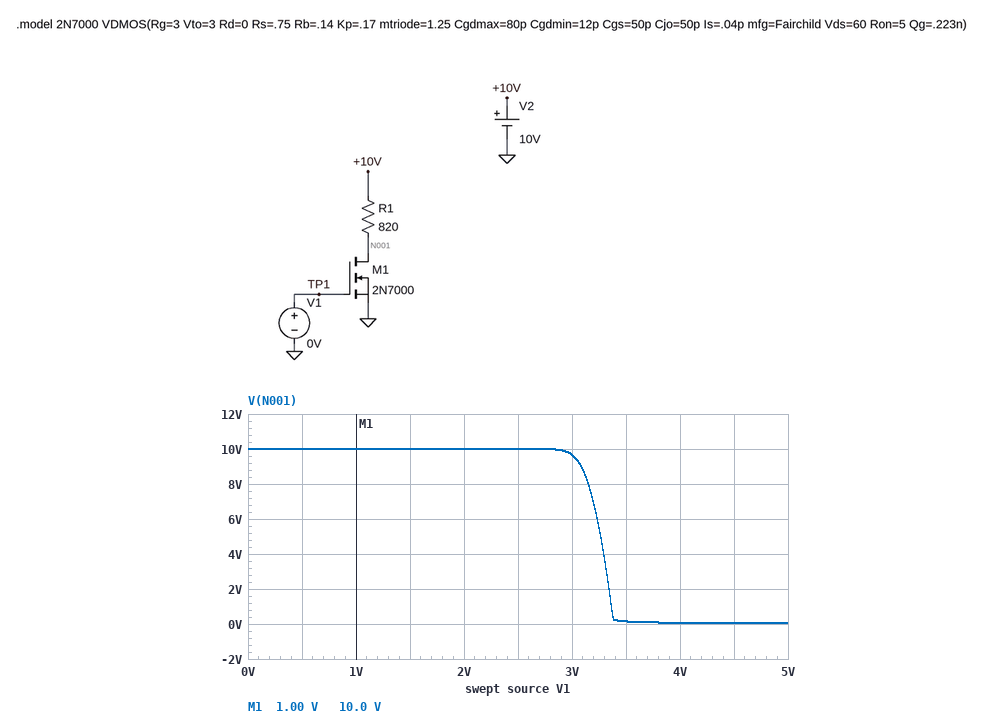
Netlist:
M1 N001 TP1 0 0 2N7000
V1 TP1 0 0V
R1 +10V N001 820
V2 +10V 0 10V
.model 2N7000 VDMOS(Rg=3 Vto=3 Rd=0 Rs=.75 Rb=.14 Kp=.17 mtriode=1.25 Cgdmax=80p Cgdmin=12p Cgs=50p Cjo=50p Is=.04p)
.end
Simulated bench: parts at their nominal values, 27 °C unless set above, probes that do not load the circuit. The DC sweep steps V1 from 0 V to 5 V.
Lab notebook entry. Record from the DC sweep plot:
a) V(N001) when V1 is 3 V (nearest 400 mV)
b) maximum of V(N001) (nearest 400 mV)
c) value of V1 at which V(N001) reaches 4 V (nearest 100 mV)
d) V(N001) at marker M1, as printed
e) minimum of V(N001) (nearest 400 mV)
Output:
9.6 V
10.0 V
3.3 V
10.0 V
0 V
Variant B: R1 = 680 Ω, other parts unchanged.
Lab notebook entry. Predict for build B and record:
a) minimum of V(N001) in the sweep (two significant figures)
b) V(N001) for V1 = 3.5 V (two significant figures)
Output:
46 mV
190 mV
